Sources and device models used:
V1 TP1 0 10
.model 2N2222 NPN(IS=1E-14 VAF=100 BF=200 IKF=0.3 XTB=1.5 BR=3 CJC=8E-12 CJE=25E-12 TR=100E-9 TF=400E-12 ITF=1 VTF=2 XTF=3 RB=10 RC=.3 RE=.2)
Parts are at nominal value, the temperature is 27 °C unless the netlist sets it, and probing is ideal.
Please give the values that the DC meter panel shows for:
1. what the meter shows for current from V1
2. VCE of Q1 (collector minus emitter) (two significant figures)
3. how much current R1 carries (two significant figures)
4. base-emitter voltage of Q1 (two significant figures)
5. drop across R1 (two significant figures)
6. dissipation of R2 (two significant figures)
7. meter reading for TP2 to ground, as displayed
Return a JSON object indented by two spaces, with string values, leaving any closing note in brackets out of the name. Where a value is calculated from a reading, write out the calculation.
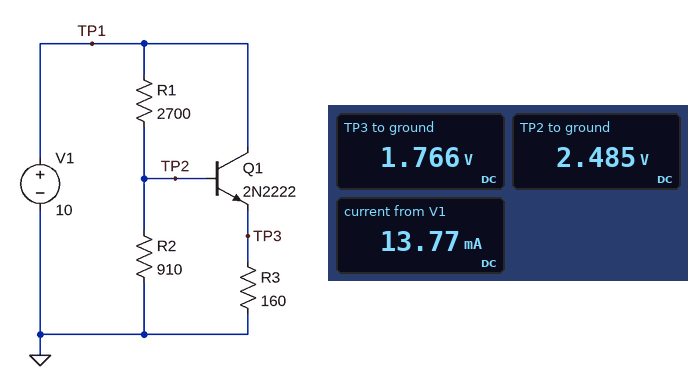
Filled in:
{
  "what the meter shows for current from V1": "13.77 mA",
  "VCE of Q1 (collector minus emitter)": "10 V - 1.766 V = 8.2 V",
  "how much current R1 carries": "(10 V - 2.485 V) / 2.7 kΩ = 2.8 mA",
  "base-emitter voltage of Q1": "2.485 V - 1.766 V = 720 mV",
  "drop across R1": "10 V - 2.485 V = 7.5 V",
  "dissipation of R2": "(2.485 V)^2 / 910 Ω = 6.8 mW",
  "meter reading for TP2 to ground, as displayed": "2.485 V"
}
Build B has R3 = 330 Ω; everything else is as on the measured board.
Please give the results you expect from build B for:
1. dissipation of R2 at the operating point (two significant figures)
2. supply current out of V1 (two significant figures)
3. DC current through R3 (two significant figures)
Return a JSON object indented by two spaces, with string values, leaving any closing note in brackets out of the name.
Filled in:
{
  "dissipation of R2 at the operating point": "6.9 mW",
  "supply current out of V1": "8.2 mA",
  "DC current through R3": "5.5 mA"
}
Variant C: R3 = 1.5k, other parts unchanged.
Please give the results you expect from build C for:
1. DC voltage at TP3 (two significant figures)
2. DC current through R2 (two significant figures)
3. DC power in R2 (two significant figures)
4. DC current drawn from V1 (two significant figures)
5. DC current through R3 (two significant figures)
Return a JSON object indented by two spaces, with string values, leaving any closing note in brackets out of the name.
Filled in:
{
  "DC voltage at TP3": "1.9 V",
  "DC current through R2": "2.8 mA",
  "DC power in R2": "7.0 mW",
  "DC current drawn from V1": "4.0 mA",
  "DC current through R3": "1.2 mA"
}
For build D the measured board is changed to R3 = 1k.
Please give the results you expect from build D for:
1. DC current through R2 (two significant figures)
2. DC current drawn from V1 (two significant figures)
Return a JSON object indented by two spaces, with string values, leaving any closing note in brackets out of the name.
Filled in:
{
  "DC current through R2": "2.8 mA",
  "DC current drawn from V1": "4.6 mA"
}
